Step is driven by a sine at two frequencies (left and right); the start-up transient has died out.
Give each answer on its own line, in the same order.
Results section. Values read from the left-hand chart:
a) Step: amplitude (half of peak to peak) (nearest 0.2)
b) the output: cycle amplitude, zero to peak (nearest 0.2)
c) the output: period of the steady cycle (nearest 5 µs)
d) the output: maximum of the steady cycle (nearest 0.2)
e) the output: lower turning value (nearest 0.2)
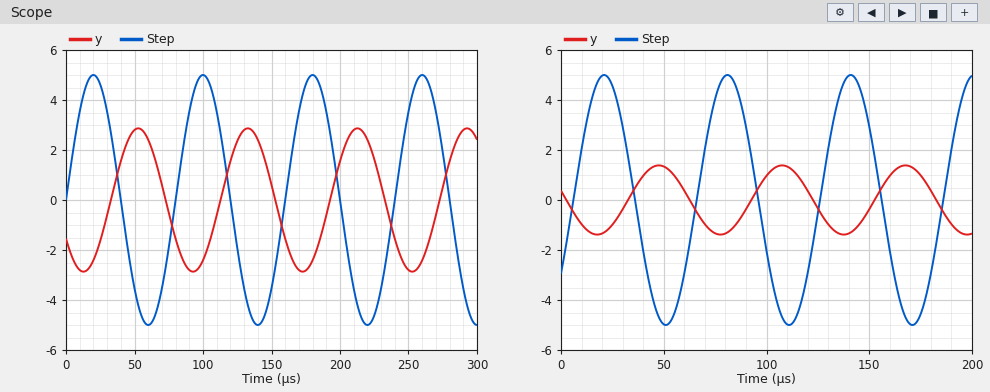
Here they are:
5.0
2.8
80 µs
2.8
-2.8
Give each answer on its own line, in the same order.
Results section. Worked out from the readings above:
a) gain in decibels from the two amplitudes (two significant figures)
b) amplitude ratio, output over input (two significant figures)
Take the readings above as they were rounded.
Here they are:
-5.0 dB
0.56
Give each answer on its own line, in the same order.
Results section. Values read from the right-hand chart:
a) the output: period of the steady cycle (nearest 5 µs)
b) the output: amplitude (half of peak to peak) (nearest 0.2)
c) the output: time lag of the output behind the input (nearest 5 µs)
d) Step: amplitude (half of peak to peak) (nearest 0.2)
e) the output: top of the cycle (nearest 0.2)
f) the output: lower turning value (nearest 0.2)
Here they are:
60 µs
1.4
25 µs
5.0
1.4
-1.4
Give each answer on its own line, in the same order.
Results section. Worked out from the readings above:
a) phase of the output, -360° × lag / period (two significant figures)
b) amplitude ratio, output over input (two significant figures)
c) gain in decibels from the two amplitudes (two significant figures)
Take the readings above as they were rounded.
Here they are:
-150°
0.28
-11 dB
